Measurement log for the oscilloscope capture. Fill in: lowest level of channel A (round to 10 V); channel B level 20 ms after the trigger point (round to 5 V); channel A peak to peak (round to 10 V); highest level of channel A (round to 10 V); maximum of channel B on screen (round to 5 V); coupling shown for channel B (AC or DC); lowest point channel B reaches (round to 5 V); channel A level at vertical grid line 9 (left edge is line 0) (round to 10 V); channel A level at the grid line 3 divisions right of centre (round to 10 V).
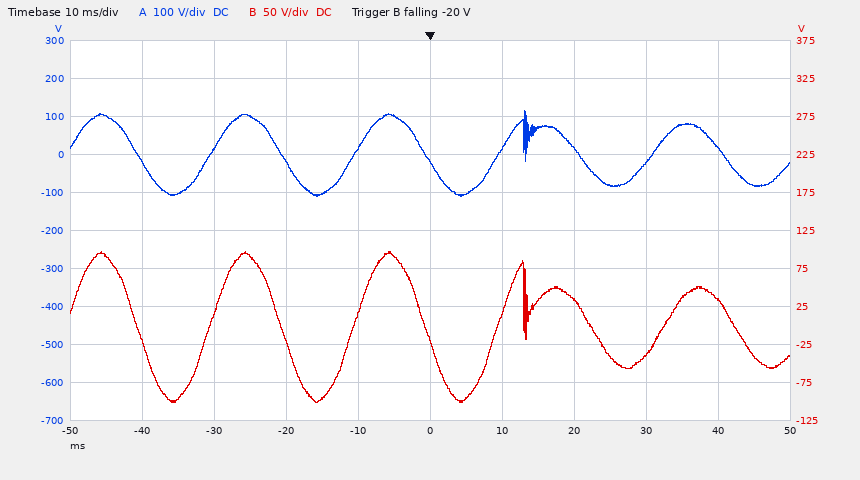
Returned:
-110 V
35 V
230 V
120 V
95 V
DC
-100 V
20 V
-20 V
